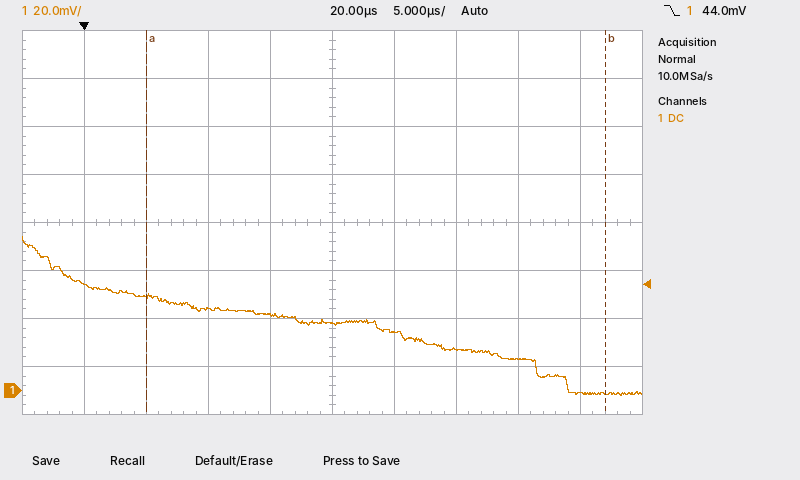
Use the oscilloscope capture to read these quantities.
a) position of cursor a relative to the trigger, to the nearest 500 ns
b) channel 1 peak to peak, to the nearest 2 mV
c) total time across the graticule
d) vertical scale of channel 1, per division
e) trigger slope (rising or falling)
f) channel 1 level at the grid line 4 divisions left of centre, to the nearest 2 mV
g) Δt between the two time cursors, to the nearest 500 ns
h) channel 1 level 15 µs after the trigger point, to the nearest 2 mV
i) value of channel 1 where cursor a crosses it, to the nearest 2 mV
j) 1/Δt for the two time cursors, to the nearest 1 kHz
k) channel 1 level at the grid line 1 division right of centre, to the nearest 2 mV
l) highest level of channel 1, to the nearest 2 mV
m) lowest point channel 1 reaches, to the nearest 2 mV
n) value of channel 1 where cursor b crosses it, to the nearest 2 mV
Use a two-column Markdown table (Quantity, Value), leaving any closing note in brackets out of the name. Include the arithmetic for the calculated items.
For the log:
| Quantity | Value |
|---|---|
| position of cursor a relative to the trigger, to the nearest 500 ns | +5.0 µs |
| channel 1 peak to peak, to the nearest 2 mV | 64 mV − (-2 mV) = 66 mV |
| total time across the graticule | 50 µs |
| vertical scale of channel 1, per division | 20 mV |
| trigger slope | falling |
| channel 1 level at the grid line 4 divisions left of centre, to the nearest 2 mV | 44 mV |
| Δt between the two time cursors, to the nearest 500 ns | 37.0 µs |
| channel 1 level 15 µs after the trigger point, to the nearest 2 mV | 32 mV |
| value of channel 1 where cursor a crosses it, to the nearest 2 mV | 40 mV |
| 1/Δt for the two time cursors, to the nearest 1 kHz | 1 / 37.0 µs ≈ 27 kHz |
| channel 1 level at the grid line 1 division right of centre, to the nearest 2 mV | 24 mV |
| highest level of channel 1, to the nearest 2 mV | 64 mV |
| lowest point channel 1 reaches, to the nearest 2 mV | -2 mV |
| value of channel 1 where cursor b crosses it, to the nearest 2 mV | -2 mV |
